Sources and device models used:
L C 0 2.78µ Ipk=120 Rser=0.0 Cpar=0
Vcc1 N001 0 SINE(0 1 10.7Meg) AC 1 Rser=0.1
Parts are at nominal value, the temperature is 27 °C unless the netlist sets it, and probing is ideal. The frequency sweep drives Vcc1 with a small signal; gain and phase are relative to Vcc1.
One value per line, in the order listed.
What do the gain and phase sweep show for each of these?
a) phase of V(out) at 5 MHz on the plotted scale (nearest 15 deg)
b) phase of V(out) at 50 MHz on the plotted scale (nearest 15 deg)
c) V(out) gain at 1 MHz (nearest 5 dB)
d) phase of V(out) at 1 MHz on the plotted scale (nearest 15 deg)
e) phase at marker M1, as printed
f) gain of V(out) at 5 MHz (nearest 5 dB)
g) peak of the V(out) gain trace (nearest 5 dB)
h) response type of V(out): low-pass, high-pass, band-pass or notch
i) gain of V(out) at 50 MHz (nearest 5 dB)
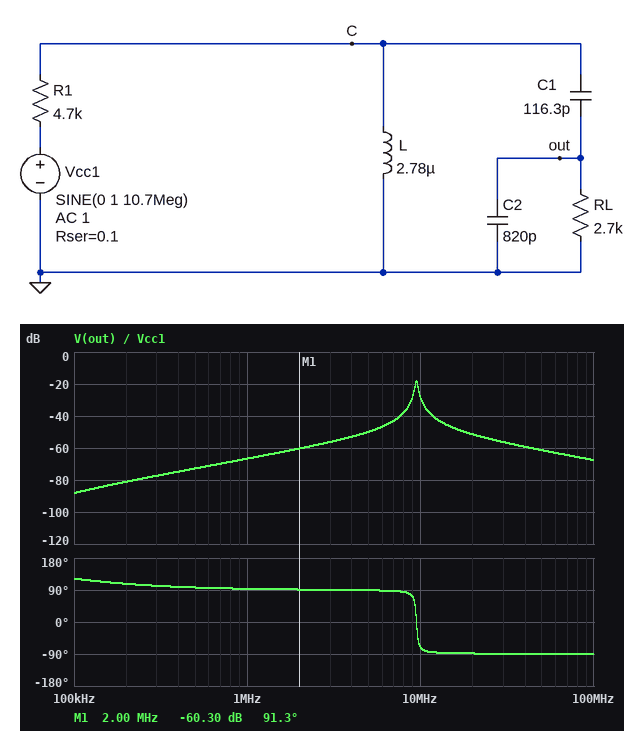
90 deg
-90 deg
-65 dB
90 deg
91.3 deg
-50 dB
-20 dB
band-pass
-60 dB
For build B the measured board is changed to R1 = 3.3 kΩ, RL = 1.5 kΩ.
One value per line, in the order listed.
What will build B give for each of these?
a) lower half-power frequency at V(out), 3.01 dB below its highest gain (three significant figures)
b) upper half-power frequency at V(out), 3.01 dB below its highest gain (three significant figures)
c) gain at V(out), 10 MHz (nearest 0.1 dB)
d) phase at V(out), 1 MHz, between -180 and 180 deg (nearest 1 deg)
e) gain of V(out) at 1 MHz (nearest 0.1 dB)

9.22 MHz
9.71 MHz
-25.9 dB
96 deg
-63.6 dB
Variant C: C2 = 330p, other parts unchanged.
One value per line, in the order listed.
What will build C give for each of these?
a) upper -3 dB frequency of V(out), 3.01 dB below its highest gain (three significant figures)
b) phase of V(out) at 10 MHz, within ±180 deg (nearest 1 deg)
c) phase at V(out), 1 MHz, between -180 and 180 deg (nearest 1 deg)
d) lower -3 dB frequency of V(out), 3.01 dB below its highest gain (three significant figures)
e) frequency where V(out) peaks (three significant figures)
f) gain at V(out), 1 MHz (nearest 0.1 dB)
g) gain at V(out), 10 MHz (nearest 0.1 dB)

10.5 MHz
54 deg
97 deg
10.1 MHz
10.3 MHz
-60.3 dB
-17.2 dB
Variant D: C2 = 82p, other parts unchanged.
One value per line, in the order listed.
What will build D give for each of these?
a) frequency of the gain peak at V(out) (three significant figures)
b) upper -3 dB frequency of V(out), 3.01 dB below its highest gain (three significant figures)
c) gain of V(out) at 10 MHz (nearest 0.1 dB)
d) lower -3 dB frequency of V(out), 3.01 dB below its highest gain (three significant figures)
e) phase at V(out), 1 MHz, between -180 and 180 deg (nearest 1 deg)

13.8 MHz
14.3 MHz
-26.8 dB
13.2 MHz
106 deg
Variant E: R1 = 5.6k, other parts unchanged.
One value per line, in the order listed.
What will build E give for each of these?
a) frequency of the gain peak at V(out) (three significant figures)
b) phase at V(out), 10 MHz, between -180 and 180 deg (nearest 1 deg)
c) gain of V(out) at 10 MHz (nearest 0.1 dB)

9.46 MHz
-74 deg
-30.0 dB
